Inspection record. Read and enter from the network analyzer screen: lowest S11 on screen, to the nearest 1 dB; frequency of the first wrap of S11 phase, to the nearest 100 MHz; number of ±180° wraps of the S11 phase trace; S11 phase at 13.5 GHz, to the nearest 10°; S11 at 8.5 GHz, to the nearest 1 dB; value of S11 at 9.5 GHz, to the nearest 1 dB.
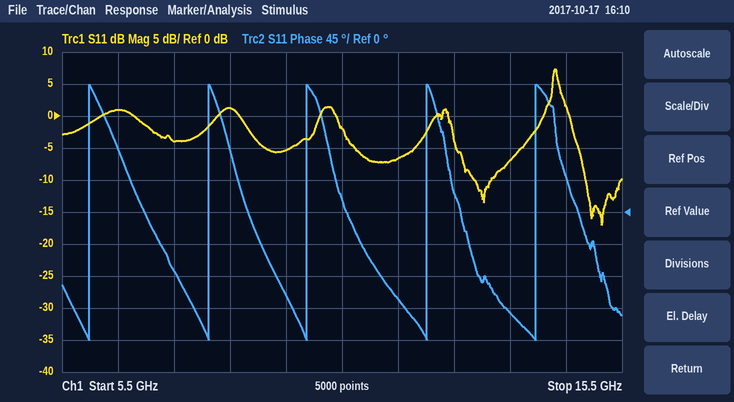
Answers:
-17 dB
6.0 GHz
5
-140°
1 dB
-5 dB
